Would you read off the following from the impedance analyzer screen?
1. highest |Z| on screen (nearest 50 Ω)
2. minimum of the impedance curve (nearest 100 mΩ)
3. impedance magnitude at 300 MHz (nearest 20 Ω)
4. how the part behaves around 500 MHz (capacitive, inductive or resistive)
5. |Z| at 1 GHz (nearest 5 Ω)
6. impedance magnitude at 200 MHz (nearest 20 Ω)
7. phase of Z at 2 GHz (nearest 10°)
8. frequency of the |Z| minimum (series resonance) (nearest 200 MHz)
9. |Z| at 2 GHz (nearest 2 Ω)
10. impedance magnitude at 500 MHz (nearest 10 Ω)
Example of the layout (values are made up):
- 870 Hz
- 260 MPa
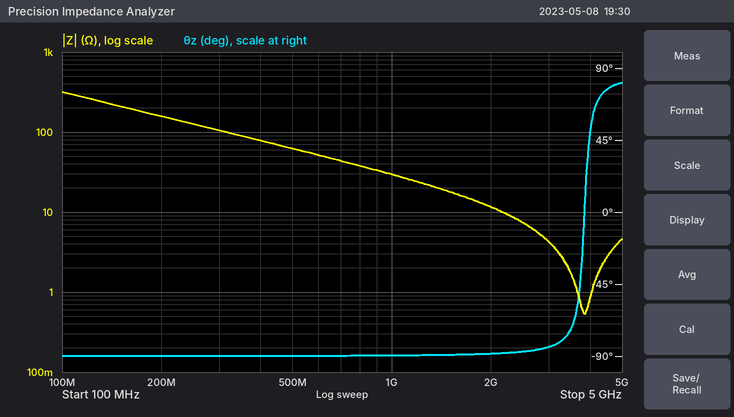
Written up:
- 300 Ω
- 500 mΩ
- 100 Ω
- capacitive
- 30 Ω
- 160 Ω
- -90°
- 3.8 GHz
- 12 Ω
- 60 Ω
